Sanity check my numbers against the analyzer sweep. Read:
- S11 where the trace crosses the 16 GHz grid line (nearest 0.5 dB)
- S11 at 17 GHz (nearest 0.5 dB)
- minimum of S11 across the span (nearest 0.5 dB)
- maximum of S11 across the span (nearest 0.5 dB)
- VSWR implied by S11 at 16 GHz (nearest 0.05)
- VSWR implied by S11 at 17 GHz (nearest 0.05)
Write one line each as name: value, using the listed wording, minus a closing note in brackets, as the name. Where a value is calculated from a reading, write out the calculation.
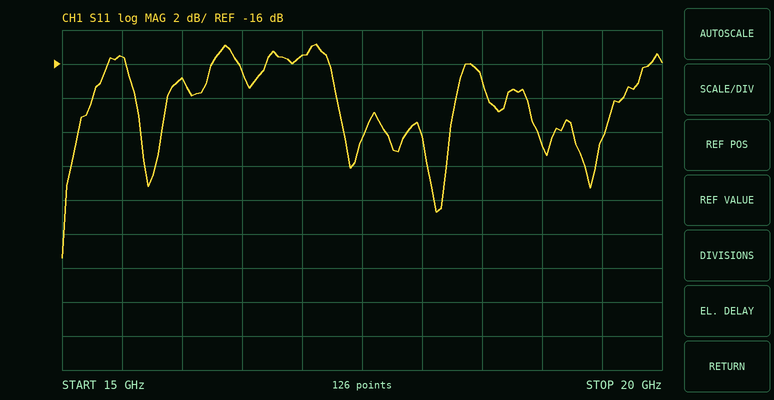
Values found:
S11 where the trace crosses the 16 GHz grid line: -17.0 dB
S11 at 17 GHz: -15.5 dB
minimum of S11 across the span: -27.5 dB
maximum of S11 across the span: -15.0 dB
VSWR implied by S11 at 16 GHz: |Γ| = 10^(-17/20) = 0.1413; VSWR = (1 + 0.1413)/(1 − 0.1413) ≈ 1.33, so 1.35 to the nearest 0.05
VSWR implied by S11 at 17 GHz: |Γ| = 10^(-15.5/20) = 0.1679; VSWR = (1 + 0.1679)/(1 − 0.1679) ≈ 1.40
